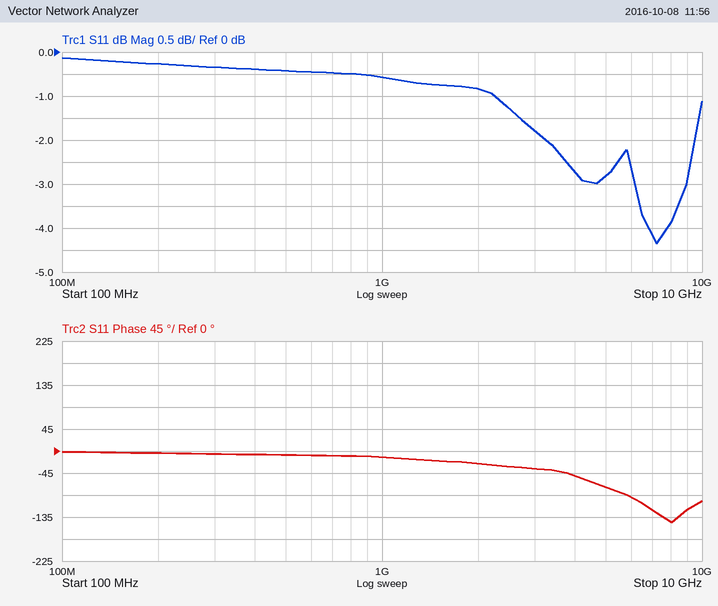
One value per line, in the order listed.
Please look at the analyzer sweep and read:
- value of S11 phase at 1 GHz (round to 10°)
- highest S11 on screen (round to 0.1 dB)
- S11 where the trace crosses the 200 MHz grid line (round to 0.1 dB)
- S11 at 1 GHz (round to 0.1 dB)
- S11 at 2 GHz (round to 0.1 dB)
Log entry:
-10°
-0.1 dB
-0.3 dB
-0.6 dB
-0.8 dB
